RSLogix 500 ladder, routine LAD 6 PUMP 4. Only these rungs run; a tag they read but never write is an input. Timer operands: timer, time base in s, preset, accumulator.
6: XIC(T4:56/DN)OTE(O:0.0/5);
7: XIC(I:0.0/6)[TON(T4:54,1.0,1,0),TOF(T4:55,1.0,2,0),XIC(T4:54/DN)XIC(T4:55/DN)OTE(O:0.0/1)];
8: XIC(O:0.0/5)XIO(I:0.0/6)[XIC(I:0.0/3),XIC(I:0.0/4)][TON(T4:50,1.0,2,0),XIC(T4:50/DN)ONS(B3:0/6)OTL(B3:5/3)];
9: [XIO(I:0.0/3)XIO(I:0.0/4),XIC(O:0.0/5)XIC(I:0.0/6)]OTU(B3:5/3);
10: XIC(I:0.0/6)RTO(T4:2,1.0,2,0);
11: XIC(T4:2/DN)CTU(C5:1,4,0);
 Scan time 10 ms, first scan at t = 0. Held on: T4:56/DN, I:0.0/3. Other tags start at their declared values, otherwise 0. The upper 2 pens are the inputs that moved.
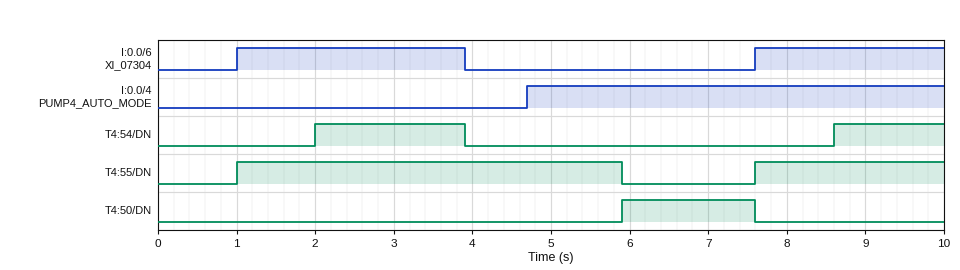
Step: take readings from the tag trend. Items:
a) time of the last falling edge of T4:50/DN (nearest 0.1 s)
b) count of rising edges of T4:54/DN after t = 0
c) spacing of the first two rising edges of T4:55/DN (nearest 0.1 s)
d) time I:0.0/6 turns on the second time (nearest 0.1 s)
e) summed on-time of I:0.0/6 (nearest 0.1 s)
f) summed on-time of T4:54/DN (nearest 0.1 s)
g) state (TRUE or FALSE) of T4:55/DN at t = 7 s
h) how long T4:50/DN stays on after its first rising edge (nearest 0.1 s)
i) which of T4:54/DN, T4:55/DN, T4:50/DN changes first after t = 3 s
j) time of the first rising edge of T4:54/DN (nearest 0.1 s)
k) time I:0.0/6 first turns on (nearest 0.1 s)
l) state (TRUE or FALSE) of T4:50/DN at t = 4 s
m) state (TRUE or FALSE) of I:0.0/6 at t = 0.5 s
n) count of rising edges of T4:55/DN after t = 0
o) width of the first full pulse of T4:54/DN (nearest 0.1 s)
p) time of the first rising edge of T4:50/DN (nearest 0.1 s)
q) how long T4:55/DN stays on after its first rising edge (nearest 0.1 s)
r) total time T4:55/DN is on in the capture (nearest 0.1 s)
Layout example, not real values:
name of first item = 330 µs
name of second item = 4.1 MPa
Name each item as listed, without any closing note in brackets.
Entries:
time of the last falling edge of T4:50/DN = 7.6 s
count of rising edges of T4:54/DN after t = 0 = 2
spacing of the first two rising edges of T4:55/DN = 6.6 s
time I:0.0/6 turns on the second time = 7.6 s
summed on-time of I:0.0/6 = 5.3 s
summed on-time of T4:54/DN = 3.3 s
state (TRUE or FALSE) of T4:55/DN at t = 7 s = FALSE
how long T4:50/DN stays on after its first rising edge = 1.7 s
which of T4:54/DN, T4:55/DN, T4:50/DN changes first after t = 3 s = T4:54/DN
time of the first rising edge of T4:54/DN = 2.0 s
time I:0.0/6 first turns on = 1.0 s
state (TRUE or FALSE) of T4:50/DN at t = 4 s = FALSE
state (TRUE or FALSE) of I:0.0/6 at t = 0.5 s = FALSE
count of rising edges of T4:55/DN after t = 0 = 2
width of the first full pulse of T4:54/DN = 1.9 s
time of the first rising edge of T4:50/DN = 5.9 s
how long T4:55/DN stays on after its first rising edge = 4.9 s
total time T4:55/DN is on in the capture = 7.3 s
